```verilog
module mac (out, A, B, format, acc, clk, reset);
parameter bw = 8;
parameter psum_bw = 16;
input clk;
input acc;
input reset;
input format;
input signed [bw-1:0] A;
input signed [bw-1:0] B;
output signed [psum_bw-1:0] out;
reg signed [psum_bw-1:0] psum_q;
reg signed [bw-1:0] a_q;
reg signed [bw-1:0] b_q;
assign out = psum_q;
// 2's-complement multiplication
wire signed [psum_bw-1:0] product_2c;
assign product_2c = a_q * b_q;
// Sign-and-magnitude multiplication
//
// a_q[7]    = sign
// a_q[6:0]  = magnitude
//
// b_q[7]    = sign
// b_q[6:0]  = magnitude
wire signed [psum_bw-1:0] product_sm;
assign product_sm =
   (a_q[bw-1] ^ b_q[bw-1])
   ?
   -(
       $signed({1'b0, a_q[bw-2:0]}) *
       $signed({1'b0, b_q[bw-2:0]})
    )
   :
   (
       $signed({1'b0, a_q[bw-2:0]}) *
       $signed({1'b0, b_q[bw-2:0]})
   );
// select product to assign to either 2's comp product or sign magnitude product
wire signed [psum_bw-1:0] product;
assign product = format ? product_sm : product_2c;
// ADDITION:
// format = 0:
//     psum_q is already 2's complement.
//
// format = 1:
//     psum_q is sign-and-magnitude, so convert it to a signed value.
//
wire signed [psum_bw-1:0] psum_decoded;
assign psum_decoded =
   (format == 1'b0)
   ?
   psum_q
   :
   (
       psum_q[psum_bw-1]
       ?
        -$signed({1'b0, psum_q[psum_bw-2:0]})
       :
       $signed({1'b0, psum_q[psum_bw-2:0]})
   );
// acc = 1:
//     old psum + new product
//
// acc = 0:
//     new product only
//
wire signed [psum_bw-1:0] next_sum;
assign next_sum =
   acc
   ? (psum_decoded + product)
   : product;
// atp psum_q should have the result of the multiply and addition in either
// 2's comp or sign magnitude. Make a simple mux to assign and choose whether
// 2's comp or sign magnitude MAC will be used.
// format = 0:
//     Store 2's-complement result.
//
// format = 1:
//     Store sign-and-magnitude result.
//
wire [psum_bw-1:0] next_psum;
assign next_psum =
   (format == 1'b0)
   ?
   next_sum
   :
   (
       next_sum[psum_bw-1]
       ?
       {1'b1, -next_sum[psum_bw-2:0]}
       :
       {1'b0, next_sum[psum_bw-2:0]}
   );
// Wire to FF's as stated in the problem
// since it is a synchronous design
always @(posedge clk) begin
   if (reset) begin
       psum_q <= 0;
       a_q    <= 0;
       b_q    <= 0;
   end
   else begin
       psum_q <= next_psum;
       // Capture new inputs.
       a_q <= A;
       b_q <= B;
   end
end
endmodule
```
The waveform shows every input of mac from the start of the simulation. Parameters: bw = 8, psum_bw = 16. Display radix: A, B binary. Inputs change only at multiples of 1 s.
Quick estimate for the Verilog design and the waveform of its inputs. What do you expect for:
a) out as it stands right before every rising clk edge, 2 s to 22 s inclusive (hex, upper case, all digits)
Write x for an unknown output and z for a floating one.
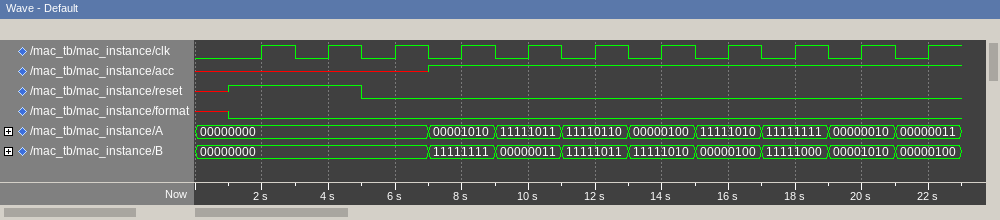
x, 0000, 0000, 0000, 0000, FFF6, FFE7, 0019, 0001, FFE9, FFF1
